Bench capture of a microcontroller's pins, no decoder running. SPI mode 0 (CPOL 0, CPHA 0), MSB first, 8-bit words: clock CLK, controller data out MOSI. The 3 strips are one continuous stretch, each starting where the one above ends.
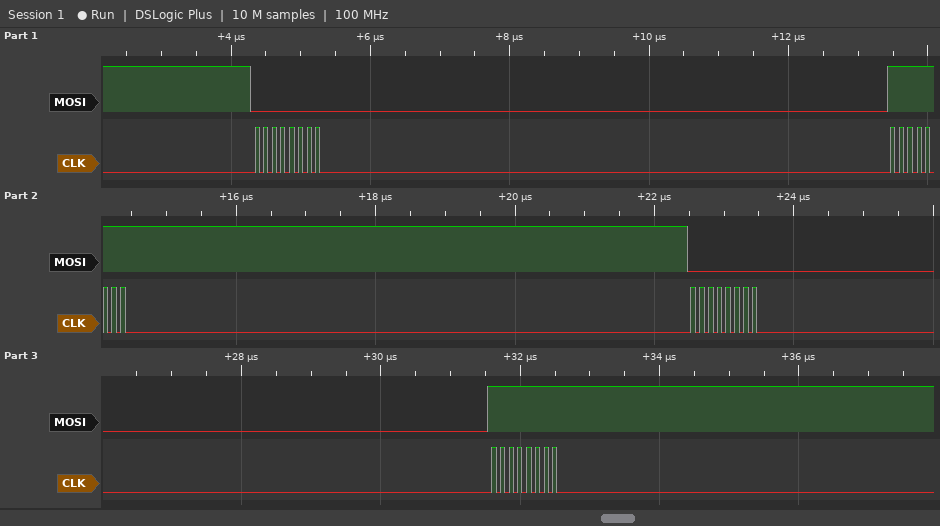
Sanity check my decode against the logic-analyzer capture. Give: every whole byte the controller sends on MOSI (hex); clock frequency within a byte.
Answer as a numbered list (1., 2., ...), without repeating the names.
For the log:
1. 00 FF 00 FF
2. 8 MHz
